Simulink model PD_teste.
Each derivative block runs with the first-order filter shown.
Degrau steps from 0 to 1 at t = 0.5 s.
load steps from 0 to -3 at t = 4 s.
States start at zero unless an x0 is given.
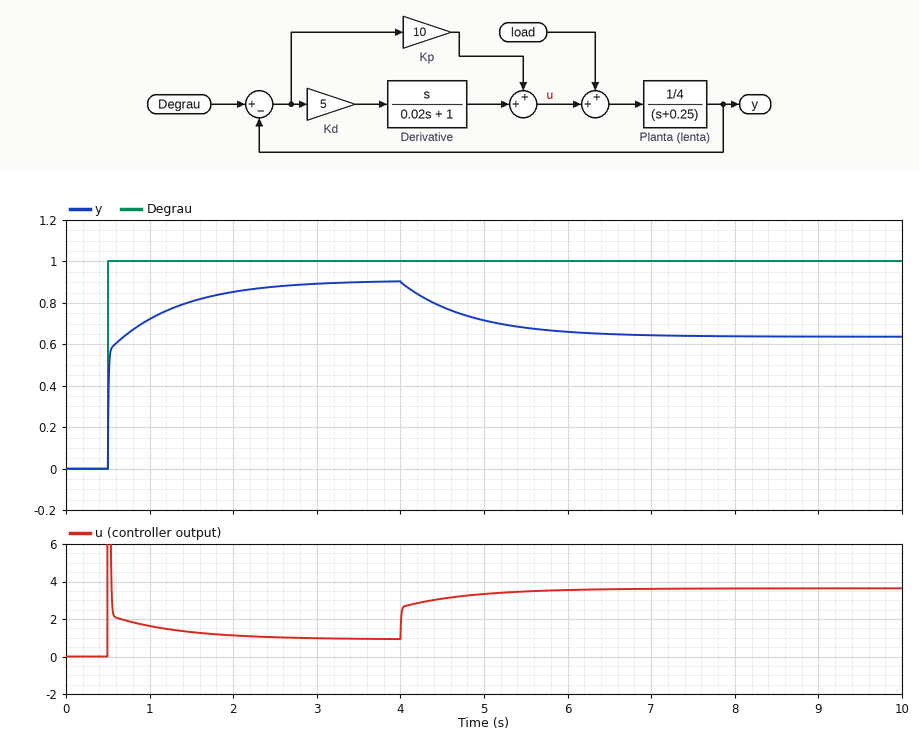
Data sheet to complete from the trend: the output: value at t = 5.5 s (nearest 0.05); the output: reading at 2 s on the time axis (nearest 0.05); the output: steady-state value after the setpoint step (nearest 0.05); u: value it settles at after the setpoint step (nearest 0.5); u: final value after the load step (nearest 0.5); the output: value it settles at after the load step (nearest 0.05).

0.70
0.85
0.90
1.0
3.5
0.65
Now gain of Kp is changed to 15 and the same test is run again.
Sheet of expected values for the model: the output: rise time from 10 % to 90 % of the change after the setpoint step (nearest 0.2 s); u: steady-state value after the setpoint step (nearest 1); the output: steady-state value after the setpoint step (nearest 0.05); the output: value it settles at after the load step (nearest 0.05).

0.8 s
1
0.95
0.75
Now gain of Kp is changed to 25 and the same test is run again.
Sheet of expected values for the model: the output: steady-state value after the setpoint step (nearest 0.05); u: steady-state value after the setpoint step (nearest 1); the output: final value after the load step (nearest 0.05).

0.95
1
0.85
